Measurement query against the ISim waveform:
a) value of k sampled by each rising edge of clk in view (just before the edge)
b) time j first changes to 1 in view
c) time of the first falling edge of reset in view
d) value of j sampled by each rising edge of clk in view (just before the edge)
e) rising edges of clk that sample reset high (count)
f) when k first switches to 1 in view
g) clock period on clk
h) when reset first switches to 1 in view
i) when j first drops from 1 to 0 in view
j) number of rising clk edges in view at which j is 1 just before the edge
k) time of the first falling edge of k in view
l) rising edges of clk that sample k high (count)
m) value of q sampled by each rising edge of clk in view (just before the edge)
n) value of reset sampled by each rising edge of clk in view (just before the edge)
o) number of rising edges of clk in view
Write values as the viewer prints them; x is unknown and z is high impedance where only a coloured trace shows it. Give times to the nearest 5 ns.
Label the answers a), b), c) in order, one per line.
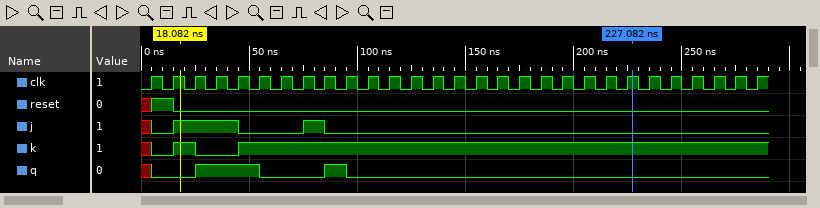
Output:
a) x 0 1 0 0 1 1 1 1 1 1 1 1 1 1 1 1 1 1 1 1 1 1 1 1 1 1 1 1
b) 15 ns
c) 15 ns
d) x 0 1 1 1 0 0 0 1 0 0 0 0 0 0 0 0 0 0 0 0 0 0 0 0 0 0 0 0
e) 1
f) 15 ns
g) 10 ns
h) 5 ns
i) 45 ns
j) 4
k) 25 ns
l) 25
m) x 0 0 1 1 1 0 0 0 1 0 0 0 0 0 0 0 0 0 0 0 0 0 0 0 0 0 0 0
n) x 1 0 0 0 0 0 0 0 0 0 0 0 0 0 0 0 0 0 0 0 0 0 0 0 0 0 0 0
o) 29
